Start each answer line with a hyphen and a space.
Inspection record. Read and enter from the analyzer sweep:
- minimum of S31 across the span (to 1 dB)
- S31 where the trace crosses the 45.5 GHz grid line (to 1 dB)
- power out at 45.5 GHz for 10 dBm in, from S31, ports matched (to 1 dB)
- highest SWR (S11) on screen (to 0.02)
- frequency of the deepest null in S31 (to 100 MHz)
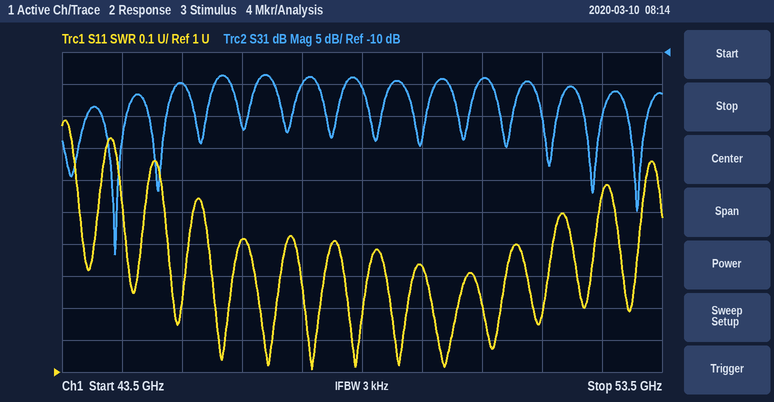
- -42 dB
- -15 dB
- -5 dBm
- 1.78
- 44.4 GHz
